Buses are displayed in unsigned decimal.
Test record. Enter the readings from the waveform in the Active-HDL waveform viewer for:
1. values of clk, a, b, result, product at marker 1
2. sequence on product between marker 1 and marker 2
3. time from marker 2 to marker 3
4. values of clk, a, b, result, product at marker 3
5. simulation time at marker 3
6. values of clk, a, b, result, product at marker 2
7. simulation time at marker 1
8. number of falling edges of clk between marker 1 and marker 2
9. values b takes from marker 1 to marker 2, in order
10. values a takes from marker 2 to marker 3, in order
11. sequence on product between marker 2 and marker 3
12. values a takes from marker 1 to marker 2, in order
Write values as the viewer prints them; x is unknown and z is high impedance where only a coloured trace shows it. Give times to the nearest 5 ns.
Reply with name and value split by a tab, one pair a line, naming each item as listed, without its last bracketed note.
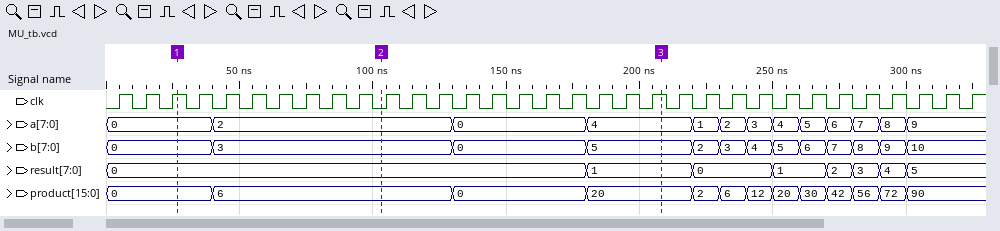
values of clk, a, b, result, product at marker 1	clk=1, a=0, b=0, result=0, product=0
sequence on product between marker 1 and marker 2	0, 6
time from marker 2 to marker 3	105 ns
values of clk, a, b, result, product at marker 3	clk=1, a=4, b=5, result=1, product=20
simulation time at marker 3	210 ns
values of clk, a, b, result, product at marker 2	clk=0, a=2, b=3, result=0, product=6
simulation time at marker 1	25 ns
number of falling edges of clk between marker 1 and marker 2	8
values b takes from marker 1 to marker 2, in order	0, 3
values a takes from marker 2 to marker 3, in order	2, 0, 4
sequence on product between marker 2 and marker 3	6, 0, 20
values a takes from marker 1 to marker 2, in order	0, 2
